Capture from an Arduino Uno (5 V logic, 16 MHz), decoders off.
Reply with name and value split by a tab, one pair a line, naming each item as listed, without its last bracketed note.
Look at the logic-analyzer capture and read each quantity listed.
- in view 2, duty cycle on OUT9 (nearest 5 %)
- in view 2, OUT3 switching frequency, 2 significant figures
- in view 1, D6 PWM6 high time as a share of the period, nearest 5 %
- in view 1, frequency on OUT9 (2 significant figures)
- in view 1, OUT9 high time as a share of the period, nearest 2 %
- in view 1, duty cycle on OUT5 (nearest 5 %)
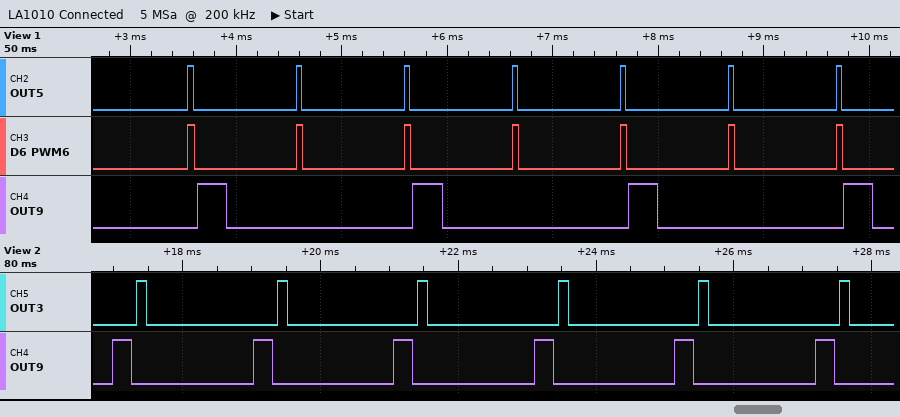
in view 2, duty cycle on OUT9	15 %
in view 2, OUT3 switching frequency, 2 significant figures	490 Hz
in view 1, D6 PWM6 high time as a share of the period, nearest 5 %	5 %
in view 1, frequency on OUT9	490 Hz
in view 1, OUT9 high time as a share of the period, nearest 2 %	14 %
in view 1, duty cycle on OUT5	5 %
